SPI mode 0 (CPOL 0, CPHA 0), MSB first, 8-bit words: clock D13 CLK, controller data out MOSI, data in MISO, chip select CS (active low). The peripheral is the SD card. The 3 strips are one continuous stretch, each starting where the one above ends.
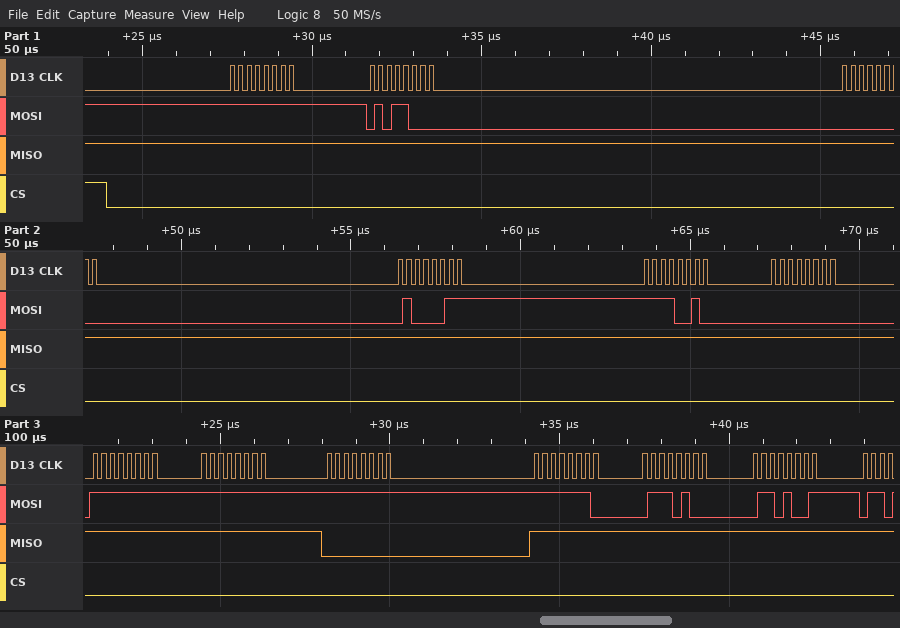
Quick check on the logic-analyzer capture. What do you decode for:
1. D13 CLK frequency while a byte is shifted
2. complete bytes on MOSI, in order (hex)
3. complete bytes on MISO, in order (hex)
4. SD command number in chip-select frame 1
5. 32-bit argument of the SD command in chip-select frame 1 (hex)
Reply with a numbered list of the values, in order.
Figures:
1. 4 MHz
2. 0xFF 0x58 0x00 0x43 0xF2 0x00 0xFF 0xFF 0xFF 0xFE 0x74 0x69
3. 0xFF 0xFF 0xFF 0xFF 0xFF 0xFF 0xFF 0xFF 0x00 0xFF 0xFF 0xFF
4. CMD24
5. 0x0043F200
